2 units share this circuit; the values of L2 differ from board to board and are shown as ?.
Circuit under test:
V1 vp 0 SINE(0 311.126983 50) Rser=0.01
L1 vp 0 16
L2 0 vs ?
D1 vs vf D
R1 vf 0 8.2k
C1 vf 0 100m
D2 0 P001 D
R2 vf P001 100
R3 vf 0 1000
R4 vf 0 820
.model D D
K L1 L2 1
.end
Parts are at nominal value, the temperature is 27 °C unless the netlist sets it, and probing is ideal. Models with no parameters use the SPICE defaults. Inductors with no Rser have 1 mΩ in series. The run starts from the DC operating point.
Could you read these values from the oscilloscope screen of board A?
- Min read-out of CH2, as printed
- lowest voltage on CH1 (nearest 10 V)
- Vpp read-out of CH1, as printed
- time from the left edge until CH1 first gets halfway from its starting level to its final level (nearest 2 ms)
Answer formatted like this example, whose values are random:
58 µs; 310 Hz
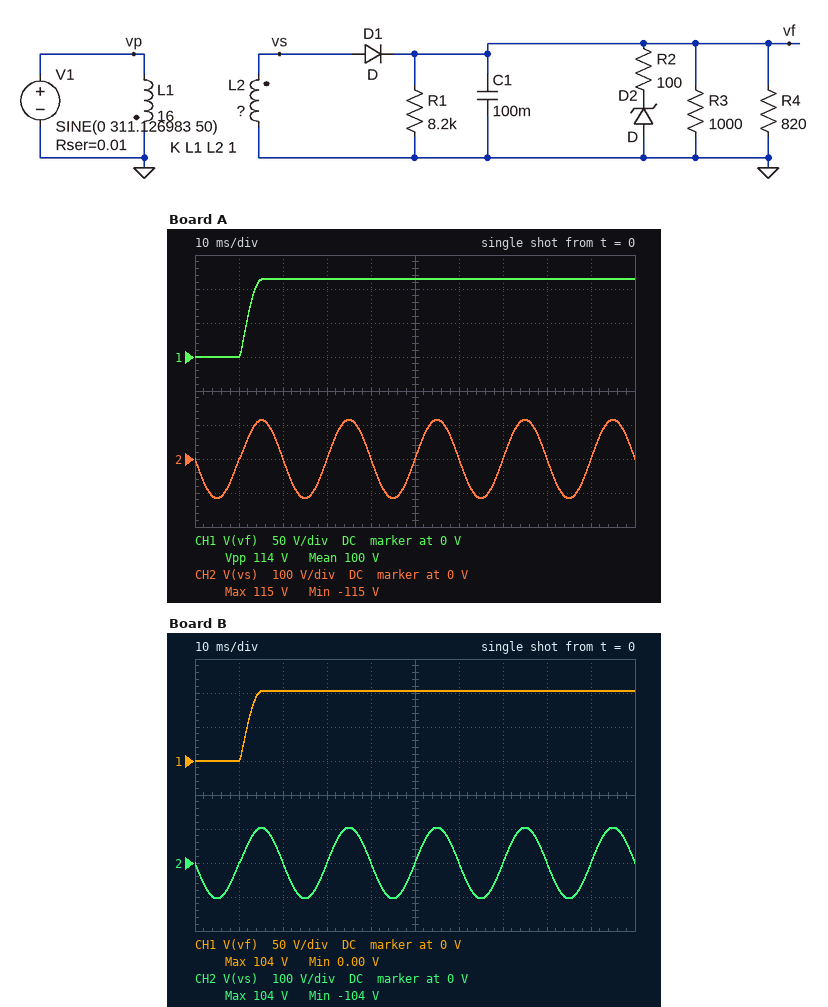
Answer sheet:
-115 V; 0 V; 114 V; 12 ms
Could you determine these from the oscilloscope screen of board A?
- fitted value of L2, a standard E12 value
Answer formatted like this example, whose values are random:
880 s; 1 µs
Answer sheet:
2.2 H
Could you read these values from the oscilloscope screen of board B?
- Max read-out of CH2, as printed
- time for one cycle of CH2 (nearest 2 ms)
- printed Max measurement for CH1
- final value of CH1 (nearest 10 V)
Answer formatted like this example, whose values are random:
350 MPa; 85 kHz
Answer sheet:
104 V; 20 ms; 104 V; 100 V
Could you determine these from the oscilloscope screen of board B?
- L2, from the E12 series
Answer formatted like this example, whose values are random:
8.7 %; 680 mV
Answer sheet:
1.8 H
